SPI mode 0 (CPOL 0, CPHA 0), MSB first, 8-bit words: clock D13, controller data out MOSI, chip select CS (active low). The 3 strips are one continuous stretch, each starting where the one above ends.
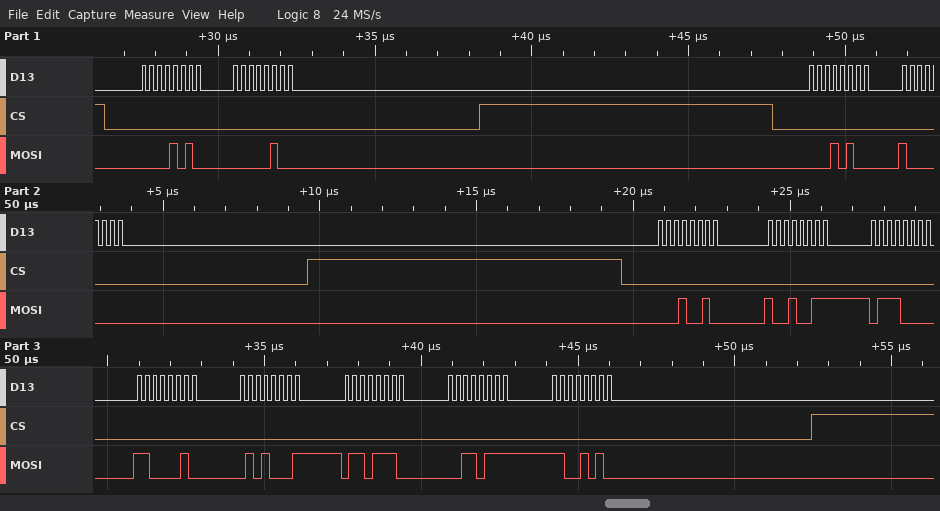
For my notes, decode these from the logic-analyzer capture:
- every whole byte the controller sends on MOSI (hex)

0A 04 14 80 12 93 70 C2 51 6E 37 CA
